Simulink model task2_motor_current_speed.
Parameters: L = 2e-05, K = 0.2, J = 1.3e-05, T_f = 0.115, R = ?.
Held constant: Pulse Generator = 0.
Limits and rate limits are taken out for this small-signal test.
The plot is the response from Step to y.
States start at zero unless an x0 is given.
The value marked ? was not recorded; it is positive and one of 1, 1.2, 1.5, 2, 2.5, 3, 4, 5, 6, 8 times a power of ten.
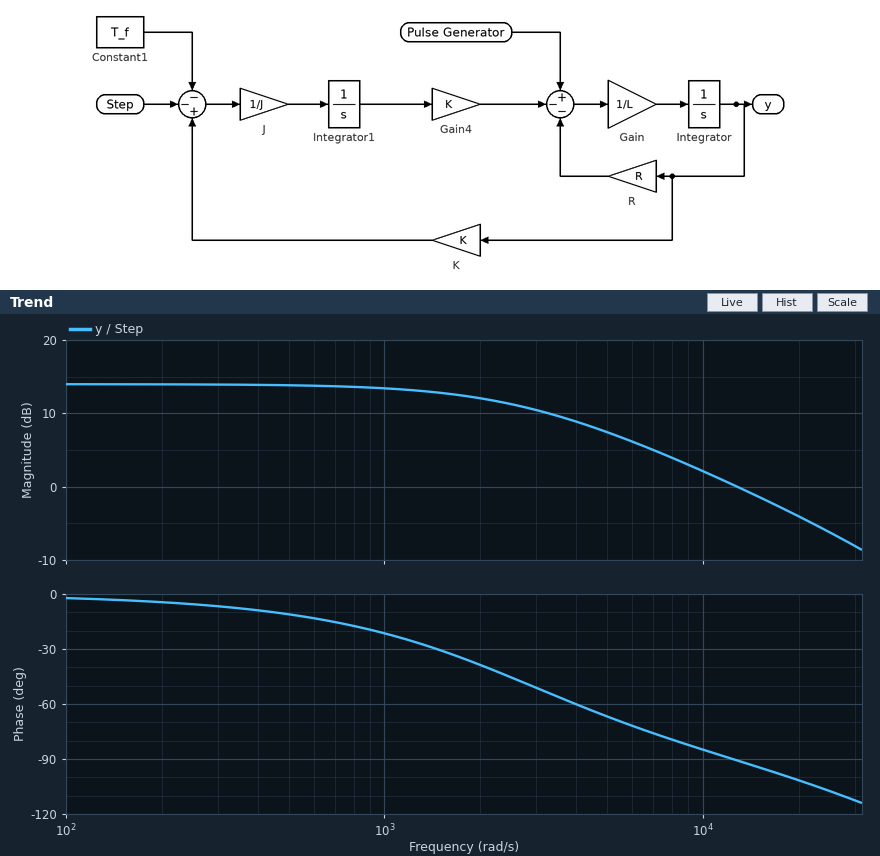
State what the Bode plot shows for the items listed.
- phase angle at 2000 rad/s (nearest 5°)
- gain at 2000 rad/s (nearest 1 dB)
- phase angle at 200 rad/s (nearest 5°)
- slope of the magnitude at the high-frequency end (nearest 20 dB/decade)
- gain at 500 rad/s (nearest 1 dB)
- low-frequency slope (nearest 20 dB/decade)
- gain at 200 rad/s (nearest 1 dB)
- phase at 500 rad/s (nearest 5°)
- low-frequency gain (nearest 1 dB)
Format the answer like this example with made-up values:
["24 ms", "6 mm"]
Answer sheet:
["-40°", "12 dB", "-5°", "-20 dB/decade", "14 dB", "0 dB/decade", "14 dB", "-10°", "14 dB"]
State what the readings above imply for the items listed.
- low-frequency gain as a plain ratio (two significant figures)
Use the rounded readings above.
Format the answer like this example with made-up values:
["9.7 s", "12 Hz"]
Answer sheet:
["5.0"]
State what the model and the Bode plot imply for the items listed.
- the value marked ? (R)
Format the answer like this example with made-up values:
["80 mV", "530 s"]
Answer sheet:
["1.2"]
